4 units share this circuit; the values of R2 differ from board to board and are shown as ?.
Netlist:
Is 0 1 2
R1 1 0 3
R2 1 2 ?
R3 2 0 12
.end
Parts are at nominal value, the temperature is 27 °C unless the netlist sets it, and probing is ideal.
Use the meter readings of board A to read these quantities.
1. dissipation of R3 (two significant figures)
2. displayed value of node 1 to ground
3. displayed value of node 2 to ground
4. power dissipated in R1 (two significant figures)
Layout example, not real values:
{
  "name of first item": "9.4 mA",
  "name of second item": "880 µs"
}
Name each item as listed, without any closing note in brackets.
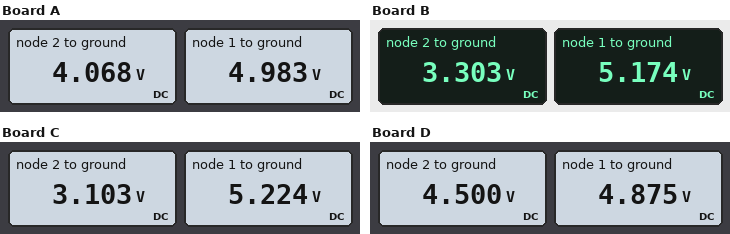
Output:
{
  "dissipation of R3": "1.4 W",
  "displayed value of node 1 to ground": "4.983 V",
  "displayed value of node 2 to ground": "4.068 V",
  "power dissipated in R1": "8.3 W"
}
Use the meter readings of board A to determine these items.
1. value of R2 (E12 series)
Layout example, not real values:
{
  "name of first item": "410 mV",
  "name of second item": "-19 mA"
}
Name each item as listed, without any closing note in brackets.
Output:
{
  "value of R2": "2.7 Ω"
}
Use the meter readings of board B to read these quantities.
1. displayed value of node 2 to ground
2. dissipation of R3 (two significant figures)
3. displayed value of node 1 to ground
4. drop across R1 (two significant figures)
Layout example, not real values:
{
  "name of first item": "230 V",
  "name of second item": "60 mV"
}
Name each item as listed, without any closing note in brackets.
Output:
{
  "displayed value of node 2 to ground": "3.303 V",
  "dissipation of R3": "910 mW",
  "displayed value of node 1 to ground": "5.174 V",
  "drop across R1": "5.2 V"
}
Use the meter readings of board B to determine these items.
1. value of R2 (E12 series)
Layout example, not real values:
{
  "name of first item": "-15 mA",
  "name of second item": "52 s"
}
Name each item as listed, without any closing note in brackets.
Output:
{
  "value of R2": "6.8 Ω"
}
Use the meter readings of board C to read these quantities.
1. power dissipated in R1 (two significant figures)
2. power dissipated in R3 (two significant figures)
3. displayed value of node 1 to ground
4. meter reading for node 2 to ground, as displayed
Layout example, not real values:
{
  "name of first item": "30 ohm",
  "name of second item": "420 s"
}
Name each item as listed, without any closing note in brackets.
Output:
{
  "power dissipated in R1": "9.1 W",
  "power dissipated in R3": "800 mW",
  "displayed value of node 1 to ground": "5.224 V",
  "meter reading for node 2 to ground, as displayed": "3.103 V"
}
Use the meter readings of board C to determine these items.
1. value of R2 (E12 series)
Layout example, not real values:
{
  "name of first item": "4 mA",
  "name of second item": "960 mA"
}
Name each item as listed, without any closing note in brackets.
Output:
{
  "value of R2": "8.2 Ω"
}
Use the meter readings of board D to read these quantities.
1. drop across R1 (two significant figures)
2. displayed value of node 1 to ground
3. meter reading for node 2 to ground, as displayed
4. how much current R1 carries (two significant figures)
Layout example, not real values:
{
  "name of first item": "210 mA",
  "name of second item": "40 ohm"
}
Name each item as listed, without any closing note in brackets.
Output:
{
  "drop across R1": "4.9 V",
  "displayed value of node 1 to ground": "4.875 V",
  "meter reading for node 2 to ground, as displayed": "4.500 V",
  "how much current R1 carries": "1.6 A"
}
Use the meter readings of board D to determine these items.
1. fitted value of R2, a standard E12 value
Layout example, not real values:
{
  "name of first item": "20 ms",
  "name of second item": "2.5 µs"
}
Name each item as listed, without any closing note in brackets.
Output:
{
  "fitted value of R2, a standard E12 value": "1 Ω"
}
